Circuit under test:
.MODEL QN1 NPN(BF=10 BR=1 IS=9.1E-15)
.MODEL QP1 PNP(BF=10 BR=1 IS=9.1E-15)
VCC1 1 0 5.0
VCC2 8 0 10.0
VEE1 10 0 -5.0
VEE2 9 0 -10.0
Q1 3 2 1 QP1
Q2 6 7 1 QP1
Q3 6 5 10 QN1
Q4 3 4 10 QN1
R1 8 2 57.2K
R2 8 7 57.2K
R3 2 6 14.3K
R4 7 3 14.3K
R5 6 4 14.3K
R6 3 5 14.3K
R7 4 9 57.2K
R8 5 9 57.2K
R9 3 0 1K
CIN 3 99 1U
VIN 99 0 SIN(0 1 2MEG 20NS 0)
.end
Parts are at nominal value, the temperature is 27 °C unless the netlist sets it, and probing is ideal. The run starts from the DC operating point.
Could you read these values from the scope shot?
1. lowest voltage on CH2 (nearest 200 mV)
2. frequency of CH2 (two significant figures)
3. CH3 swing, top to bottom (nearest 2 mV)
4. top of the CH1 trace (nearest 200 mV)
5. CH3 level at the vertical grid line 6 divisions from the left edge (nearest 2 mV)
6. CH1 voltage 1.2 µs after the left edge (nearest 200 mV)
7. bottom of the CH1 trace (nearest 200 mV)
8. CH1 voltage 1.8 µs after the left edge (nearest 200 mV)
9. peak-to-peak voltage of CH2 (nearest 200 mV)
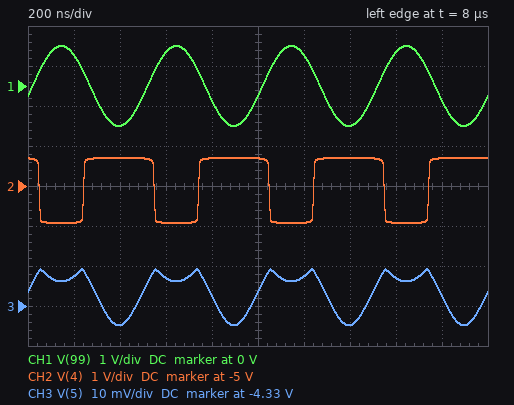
-6.0 V
2.0 MHz
14 mV
1.0 V
-4.322 V
800 mV
-1.0 V
-400 mV
1.6 V
